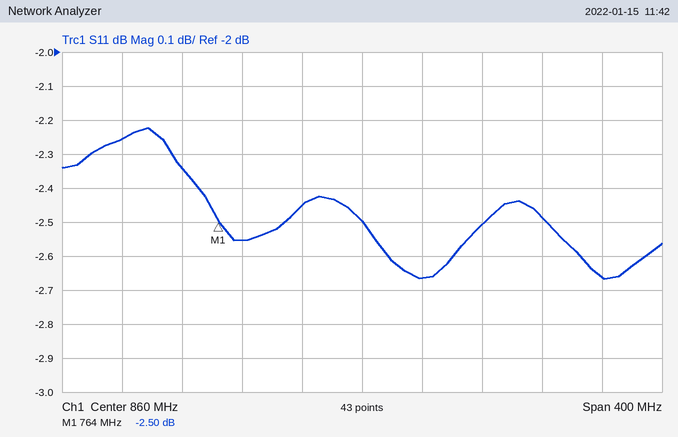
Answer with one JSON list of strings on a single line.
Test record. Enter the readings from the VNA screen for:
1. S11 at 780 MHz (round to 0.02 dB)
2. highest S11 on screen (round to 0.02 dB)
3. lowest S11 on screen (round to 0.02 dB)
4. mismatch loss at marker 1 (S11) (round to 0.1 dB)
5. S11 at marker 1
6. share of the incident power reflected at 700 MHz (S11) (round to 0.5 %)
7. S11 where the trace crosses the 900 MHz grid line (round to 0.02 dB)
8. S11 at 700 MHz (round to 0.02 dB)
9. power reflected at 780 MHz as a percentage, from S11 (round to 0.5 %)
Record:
["-2.56 dB", "-2.22 dB", "-2.66 dB", "3.6 dB", "-2.50 dB", "59.5 %", "-2.66 dB", "-2.26 dB", "55.5 %"]
